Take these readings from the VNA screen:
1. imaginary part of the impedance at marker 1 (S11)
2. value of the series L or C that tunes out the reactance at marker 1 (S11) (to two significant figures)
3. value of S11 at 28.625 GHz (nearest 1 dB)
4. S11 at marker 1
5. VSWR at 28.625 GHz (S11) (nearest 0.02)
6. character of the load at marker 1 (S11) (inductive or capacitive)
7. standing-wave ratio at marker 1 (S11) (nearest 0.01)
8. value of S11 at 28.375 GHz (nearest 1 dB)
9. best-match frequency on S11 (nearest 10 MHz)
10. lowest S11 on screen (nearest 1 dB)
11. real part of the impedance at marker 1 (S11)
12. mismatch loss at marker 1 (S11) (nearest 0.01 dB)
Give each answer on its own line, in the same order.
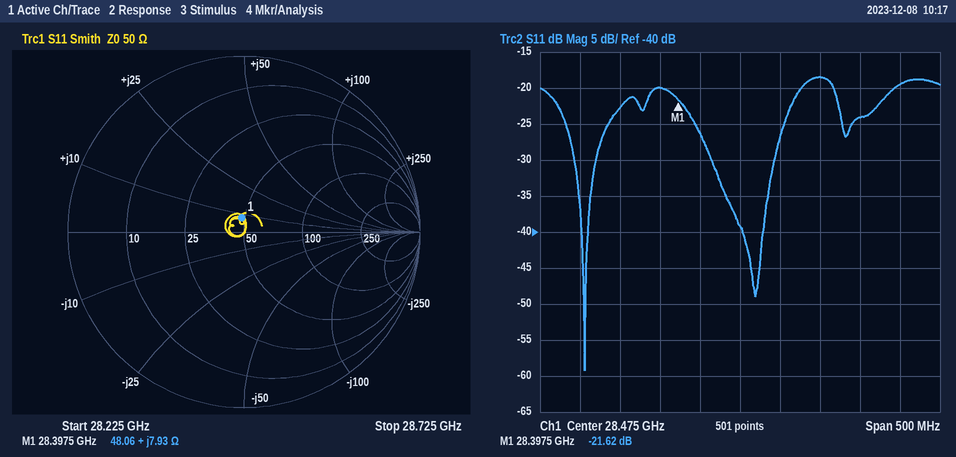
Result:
+7.93 Ω
710 fF
-24 dB
-21.62 dB
1.14
inductive
1.18
-20 dB
28.28 GHz
-59 dB
48.06 Ω
0.03 dB
